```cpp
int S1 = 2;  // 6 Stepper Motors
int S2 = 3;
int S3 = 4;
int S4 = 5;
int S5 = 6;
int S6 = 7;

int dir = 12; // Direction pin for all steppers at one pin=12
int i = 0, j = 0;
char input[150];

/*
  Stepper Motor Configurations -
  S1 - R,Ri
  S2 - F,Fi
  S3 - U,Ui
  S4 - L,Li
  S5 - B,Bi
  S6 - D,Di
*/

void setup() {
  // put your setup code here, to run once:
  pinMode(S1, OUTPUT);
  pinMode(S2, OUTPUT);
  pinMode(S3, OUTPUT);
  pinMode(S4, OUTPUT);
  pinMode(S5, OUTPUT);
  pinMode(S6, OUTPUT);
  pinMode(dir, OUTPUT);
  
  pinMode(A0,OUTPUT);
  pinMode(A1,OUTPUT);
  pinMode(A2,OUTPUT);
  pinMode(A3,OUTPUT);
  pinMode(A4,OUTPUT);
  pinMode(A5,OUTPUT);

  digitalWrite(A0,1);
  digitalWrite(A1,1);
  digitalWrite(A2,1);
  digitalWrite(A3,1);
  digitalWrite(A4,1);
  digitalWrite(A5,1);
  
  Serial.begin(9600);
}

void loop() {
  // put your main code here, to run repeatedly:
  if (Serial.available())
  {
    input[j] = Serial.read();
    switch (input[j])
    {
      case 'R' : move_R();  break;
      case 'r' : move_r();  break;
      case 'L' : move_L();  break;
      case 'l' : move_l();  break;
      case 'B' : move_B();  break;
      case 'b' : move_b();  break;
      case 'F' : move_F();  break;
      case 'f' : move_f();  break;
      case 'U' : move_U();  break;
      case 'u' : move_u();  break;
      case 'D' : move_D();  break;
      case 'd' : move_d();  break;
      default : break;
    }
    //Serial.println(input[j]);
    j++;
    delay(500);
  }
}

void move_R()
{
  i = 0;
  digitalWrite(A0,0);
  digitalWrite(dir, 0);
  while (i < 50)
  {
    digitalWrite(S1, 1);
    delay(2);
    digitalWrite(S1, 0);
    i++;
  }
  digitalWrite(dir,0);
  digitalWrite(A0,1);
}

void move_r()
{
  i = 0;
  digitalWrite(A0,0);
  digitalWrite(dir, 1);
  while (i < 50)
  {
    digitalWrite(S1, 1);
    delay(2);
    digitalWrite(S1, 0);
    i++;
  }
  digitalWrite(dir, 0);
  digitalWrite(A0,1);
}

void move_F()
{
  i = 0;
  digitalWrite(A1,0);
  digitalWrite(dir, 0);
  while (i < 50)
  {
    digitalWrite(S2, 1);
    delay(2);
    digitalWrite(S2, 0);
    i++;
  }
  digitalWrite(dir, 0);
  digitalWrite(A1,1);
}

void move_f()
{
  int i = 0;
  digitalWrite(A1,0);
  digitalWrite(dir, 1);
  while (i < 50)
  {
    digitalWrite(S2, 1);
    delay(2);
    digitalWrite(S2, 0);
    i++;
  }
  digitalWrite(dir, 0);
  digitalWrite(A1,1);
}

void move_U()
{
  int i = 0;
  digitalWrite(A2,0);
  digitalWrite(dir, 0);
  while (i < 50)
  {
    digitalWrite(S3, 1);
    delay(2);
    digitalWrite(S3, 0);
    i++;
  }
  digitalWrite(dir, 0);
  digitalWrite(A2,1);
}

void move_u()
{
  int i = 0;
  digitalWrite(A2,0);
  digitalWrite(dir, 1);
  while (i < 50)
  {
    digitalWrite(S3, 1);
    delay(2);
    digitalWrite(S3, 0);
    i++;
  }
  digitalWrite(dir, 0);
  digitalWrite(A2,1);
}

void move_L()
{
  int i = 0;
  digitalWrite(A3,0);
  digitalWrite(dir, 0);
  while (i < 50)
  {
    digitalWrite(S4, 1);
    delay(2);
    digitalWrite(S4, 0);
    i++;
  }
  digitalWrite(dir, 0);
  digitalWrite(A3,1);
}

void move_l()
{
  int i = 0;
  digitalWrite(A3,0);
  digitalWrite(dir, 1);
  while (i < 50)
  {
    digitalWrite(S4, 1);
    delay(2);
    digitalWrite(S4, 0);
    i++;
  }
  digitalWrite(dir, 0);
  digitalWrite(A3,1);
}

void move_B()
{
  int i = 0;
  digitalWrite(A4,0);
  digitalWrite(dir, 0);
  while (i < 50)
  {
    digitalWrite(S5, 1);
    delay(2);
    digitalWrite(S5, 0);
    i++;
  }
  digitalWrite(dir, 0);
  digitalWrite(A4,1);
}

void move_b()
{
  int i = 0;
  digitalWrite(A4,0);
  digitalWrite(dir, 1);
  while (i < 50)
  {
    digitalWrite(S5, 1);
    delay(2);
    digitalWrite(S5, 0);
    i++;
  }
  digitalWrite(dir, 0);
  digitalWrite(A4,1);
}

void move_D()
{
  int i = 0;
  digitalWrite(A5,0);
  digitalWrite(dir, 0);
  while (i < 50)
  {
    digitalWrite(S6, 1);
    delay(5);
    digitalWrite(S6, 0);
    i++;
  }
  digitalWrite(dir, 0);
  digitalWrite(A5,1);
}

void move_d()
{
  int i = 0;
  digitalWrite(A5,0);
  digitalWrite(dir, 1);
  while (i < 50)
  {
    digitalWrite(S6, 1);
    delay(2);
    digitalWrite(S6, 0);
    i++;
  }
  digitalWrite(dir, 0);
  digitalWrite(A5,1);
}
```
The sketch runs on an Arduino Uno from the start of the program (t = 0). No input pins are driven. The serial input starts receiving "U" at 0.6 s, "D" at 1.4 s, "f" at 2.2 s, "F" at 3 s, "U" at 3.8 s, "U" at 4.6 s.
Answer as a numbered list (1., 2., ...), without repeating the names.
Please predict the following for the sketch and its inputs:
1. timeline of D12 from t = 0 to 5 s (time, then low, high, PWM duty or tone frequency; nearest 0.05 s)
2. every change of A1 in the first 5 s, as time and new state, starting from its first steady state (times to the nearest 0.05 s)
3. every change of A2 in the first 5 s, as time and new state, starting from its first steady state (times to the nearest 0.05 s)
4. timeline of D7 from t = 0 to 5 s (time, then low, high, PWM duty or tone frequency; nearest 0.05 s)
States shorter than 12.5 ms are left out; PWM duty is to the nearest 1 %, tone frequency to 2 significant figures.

1. 0 s low; 2.2 s high; 2.3 s low
2. 0 s high; 2.2 s low; 2.3 s high; 3 s low; 3.1 s high
3. 0 s high; 0.6 s low; 0.7 s high; 3.8 s low; 3.9 s high; 4.6 s low; 4.7 s high
4. 0 s low; 1.4 s tone 200 Hz; 1.65 s low
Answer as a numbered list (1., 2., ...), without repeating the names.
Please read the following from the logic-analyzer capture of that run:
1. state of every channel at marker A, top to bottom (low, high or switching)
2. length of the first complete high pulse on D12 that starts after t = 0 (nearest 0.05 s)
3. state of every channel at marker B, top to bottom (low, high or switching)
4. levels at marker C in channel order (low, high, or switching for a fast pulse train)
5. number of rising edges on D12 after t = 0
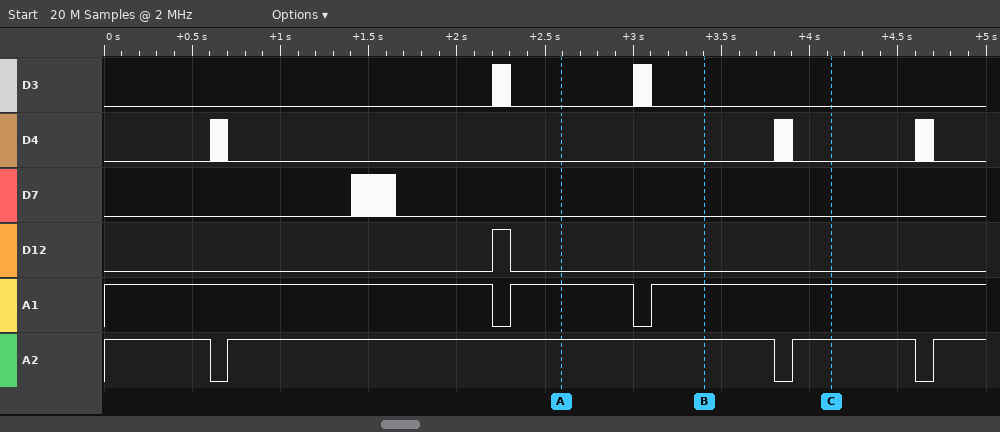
1. D3 low, D4 low, D7 low, D12 low, A1 high, A2 high
2. 0.10 s
3. D3 low, D4 low, D7 low, D12 low, A1 high, A2 high
4. D3 low, D4 low, D7 low, D12 low, A1 high, A2 high
5. 1
